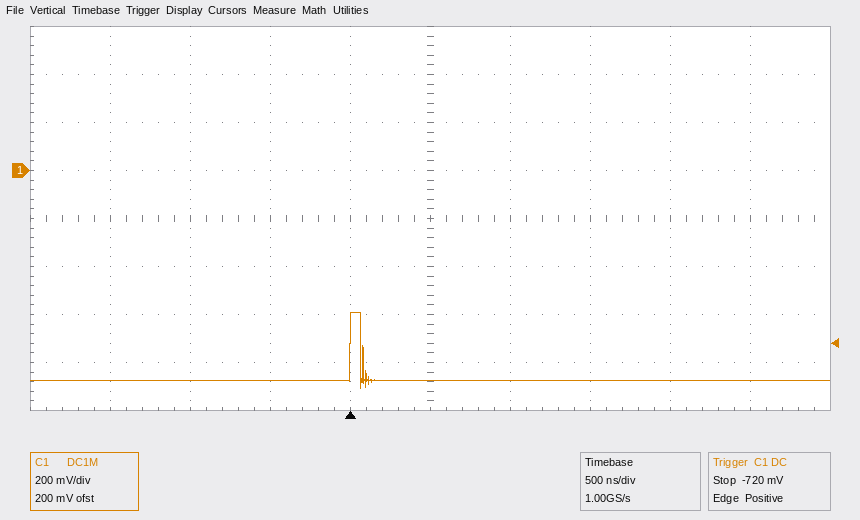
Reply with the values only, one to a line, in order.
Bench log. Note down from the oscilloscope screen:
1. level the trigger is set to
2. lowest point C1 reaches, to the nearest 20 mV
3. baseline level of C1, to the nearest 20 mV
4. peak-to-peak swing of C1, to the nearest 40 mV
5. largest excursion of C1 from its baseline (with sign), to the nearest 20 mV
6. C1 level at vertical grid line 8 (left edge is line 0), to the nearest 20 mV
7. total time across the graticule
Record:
-720 mV
-900 mV
-880 mV
320 mV
+280 mV
-880 mV
5 µs
